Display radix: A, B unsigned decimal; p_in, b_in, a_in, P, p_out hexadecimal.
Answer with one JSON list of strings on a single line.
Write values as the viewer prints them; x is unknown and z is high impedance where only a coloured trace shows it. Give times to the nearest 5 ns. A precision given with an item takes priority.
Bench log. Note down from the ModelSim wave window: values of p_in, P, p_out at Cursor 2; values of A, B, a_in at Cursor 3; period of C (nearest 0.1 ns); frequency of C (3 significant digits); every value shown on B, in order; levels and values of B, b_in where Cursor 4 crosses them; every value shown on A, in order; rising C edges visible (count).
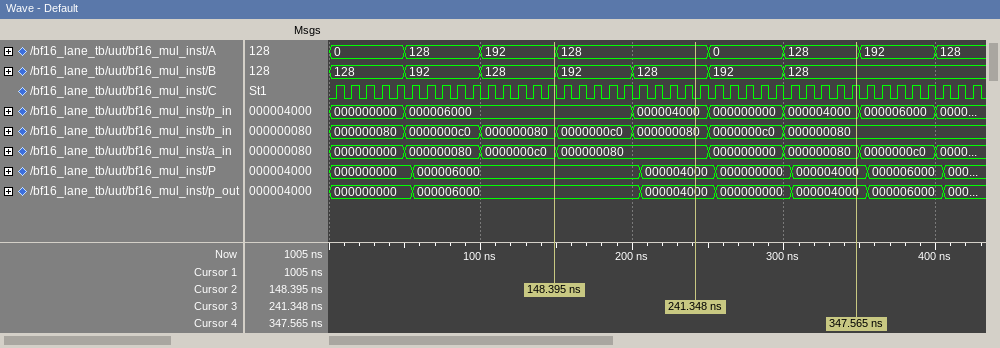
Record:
["p_in=000006000, P=000006000, p_out=000006000", "A=128, B=128, a_in=000000080", "10 ns", "100 MHz", "128, 192, 128, 192, 128, 192, 128", "B=128, b_in=000000080", "0, 128, 192, 128, 0, 128, 192, 128", "43"]
